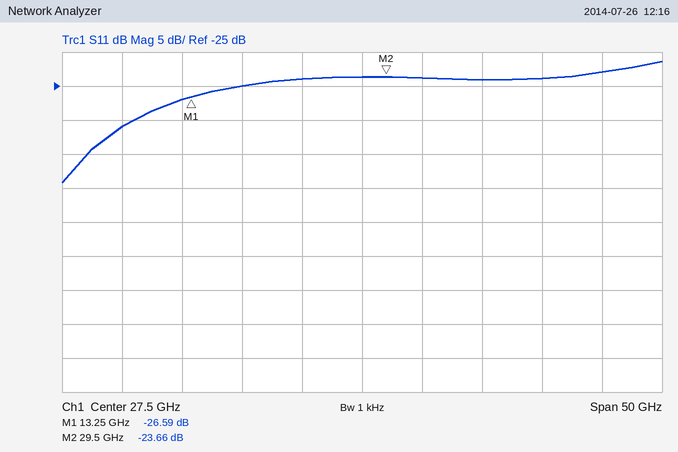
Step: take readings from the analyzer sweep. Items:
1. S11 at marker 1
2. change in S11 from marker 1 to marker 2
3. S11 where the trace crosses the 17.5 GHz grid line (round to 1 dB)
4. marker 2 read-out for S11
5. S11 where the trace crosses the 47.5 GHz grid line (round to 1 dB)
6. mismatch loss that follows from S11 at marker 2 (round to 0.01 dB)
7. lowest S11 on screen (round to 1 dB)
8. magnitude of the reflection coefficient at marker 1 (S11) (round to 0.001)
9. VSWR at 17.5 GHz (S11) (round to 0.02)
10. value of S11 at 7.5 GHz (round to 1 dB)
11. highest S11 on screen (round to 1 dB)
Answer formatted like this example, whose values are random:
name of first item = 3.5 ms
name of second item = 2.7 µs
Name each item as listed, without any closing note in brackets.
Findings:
S11 at marker 1 = -26.59 dB
change in S11 from marker 1 to marker 2 = 2.93 dB
S11 where the trace crosses the 17.5 GHz grid line = -25 dB
marker 2 read-out for S11 = -23.66 dB
S11 where the trace crosses the 47.5 GHz grid line = -23 dB
mismatch loss that follows from S11 at marker 2 = 0.02 dB
lowest S11 on screen = -39 dB
magnitude of the reflection coefficient at marker 1 (S11) = 0.047
VSWR at 17.5 GHz (S11) = 1.12
value of S11 at 7.5 GHz = -31 dB
highest S11 on screen = -21 dB
